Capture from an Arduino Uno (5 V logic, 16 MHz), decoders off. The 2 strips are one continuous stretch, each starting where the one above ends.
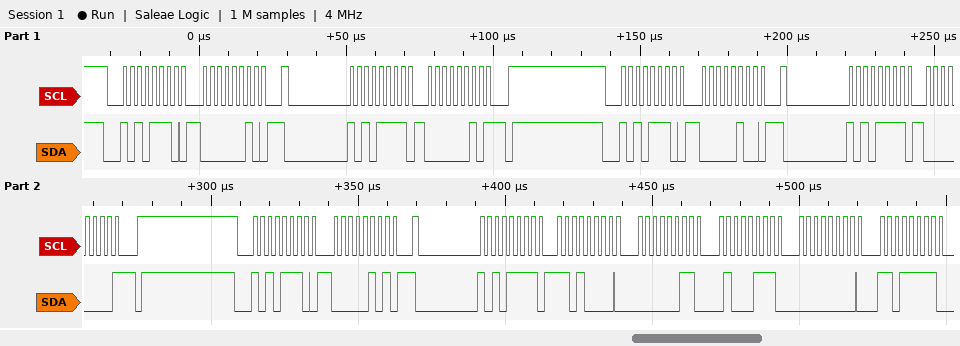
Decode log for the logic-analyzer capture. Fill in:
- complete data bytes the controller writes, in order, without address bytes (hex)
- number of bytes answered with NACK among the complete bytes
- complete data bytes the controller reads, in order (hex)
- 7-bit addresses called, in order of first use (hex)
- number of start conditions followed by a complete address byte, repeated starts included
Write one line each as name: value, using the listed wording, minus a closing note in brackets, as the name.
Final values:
complete data bytes the controller writes, in order, without address bytes: 02 04 05
number of bytes answered with NACK among the complete bytes: 2
complete data bytes the controller reads, in order: 02 00 D0 03 47 00 DF
7-bit addresses called, in order of first use: 0x57
number of start conditions followed by a complete address byte, repeated starts included: 6
